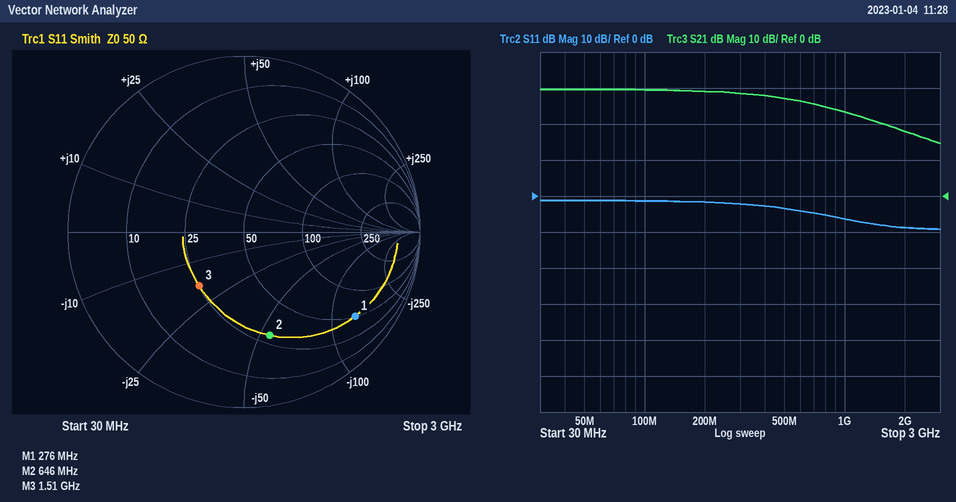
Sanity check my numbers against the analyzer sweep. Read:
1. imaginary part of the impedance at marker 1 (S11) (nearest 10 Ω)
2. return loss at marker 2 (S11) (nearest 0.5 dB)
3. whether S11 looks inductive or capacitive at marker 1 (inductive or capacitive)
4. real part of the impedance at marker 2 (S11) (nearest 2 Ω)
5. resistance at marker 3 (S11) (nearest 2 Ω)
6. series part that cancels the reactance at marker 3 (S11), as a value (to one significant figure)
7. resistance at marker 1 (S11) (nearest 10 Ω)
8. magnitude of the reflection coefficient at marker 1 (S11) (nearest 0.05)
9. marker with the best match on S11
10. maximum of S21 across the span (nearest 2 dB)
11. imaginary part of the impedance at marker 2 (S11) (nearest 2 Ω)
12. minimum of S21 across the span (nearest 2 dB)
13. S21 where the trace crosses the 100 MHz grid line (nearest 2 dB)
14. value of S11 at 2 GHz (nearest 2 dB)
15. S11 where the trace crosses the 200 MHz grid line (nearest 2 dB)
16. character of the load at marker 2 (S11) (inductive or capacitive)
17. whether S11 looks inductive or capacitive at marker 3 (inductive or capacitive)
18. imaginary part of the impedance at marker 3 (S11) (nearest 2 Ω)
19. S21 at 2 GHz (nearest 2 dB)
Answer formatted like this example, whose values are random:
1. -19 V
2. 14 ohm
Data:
1. -130 Ω
2. 4.5 dB
3. capacitive
4. 30 Ω
5. 26 Ω
6. 2 nH
7. 50 Ω
8. 0.80
9. marker 3
10. 30 dB
11. -54 Ω
12. 14 dB
13. 30 dB
14. -8 dB
15. -2 dB
16. capacitive
17. capacitive
18. -18 Ω
19. 18 dB
